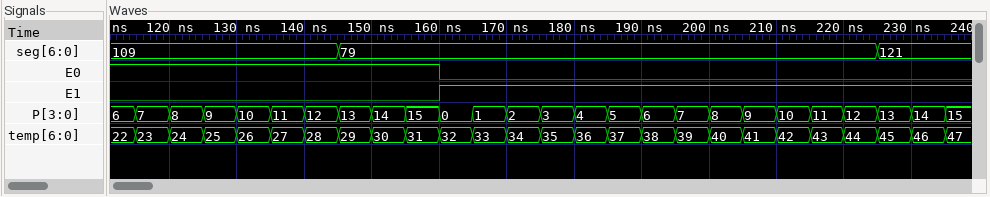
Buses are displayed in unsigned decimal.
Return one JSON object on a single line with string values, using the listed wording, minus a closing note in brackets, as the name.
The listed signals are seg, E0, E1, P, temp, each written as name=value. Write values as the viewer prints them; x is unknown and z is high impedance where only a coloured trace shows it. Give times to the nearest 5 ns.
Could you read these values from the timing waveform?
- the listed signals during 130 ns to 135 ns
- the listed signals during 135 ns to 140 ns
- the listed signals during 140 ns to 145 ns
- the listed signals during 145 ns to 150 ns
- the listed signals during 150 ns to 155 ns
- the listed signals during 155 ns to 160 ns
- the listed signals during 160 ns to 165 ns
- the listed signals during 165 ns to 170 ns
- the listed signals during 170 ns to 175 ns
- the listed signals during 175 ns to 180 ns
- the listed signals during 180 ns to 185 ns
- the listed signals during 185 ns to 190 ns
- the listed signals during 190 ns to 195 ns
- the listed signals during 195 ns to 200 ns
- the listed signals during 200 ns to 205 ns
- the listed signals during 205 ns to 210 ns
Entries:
{"the listed signals during 130 ns to 135 ns": "seg=109, E0=1, E1=0, P=10, temp=26", "the listed signals during 135 ns to 140 ns": "seg=109, E0=1, E1=0, P=11, temp=27", "the listed signals during 140 ns to 145 ns": "seg=109, E0=1, E1=0, P=12, temp=28", "the listed signals during 145 ns to 150 ns": "seg=79, E0=1, E1=0, P=13, temp=29", "the listed signals during 150 ns to 155 ns": "seg=79, E0=1, E1=0, P=14, temp=30", "the listed signals during 155 ns to 160 ns": "seg=79, E0=1, E1=0, P=15, temp=31", "the listed signals during 160 ns to 165 ns": "seg=79, E0=0, E1=1, P=0, temp=32", "the listed signals during 165 ns to 170 ns": "seg=79, E0=0, E1=1, P=1, temp=33", "the listed signals during 170 ns to 175 ns": "seg=79, E0=0, E1=1, P=2, temp=34", "the listed signals during 175 ns to 180 ns": "seg=79, E0=0, E1=1, P=3, temp=35", "the listed signals during 180 ns to 185 ns": "seg=79, E0=0, E1=1, P=4, temp=36", "the listed signals during 185 ns to 190 ns": "seg=79, E0=0, E1=1, P=5, temp=37", "the listed signals during 190 ns to 195 ns": "seg=79, E0=0, E1=1, P=6, temp=38", "the listed signals during 195 ns to 200 ns": "seg=79, E0=0, E1=1, P=7, temp=39", "the listed signals during 200 ns to 205 ns": "seg=79, E0=0, E1=1, P=8, temp=40", "the listed signals during 205 ns to 210 ns": "seg=79, E0=0, E1=1, P=9, temp=41"}
